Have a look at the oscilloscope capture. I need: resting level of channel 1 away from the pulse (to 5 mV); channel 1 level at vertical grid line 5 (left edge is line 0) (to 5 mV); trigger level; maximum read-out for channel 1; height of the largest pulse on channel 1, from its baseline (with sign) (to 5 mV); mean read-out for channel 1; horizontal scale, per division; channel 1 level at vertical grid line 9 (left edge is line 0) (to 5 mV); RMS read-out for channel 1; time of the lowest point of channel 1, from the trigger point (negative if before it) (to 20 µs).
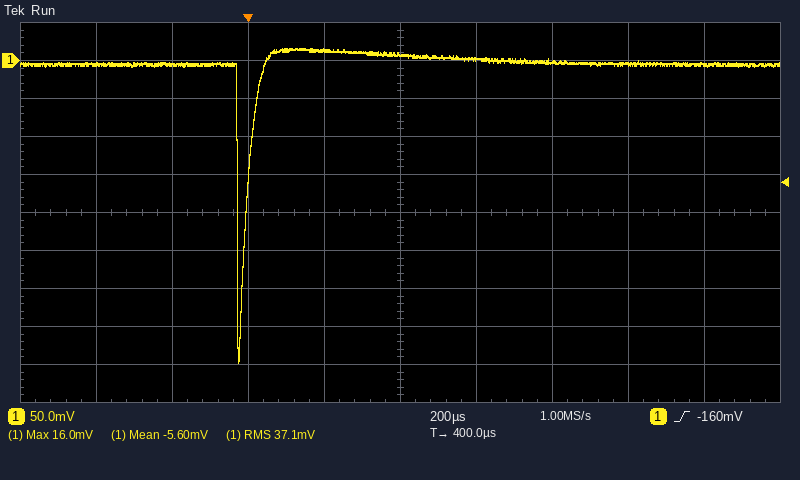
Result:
-5 mV
10 mV
-160 mV
16.0 mV
-395 mV
-5.60 mV
200 µs
-5 mV
37.1 mV
-20 µs
